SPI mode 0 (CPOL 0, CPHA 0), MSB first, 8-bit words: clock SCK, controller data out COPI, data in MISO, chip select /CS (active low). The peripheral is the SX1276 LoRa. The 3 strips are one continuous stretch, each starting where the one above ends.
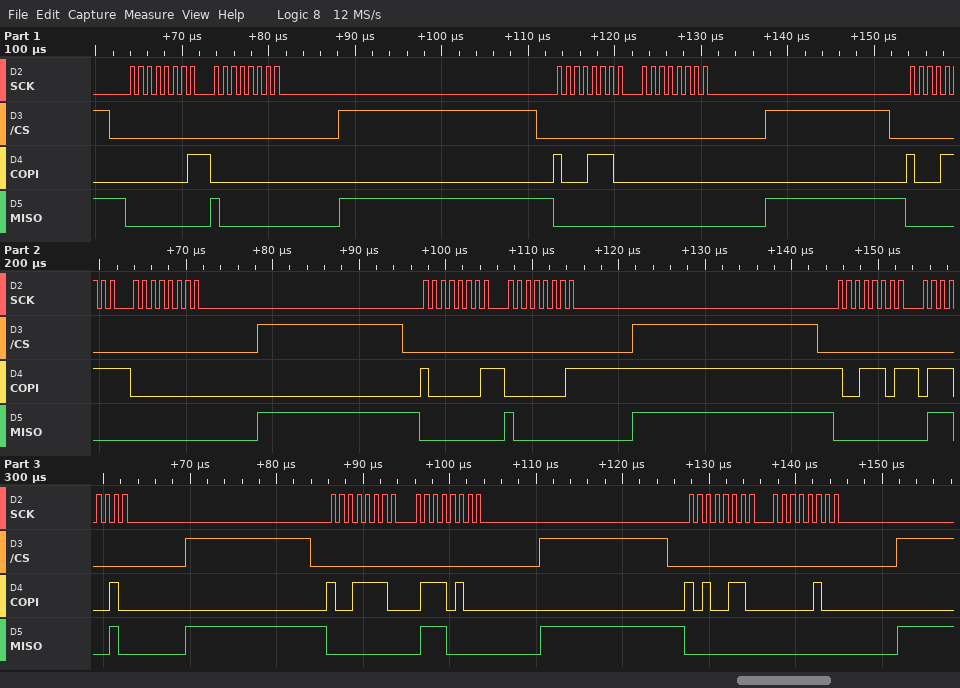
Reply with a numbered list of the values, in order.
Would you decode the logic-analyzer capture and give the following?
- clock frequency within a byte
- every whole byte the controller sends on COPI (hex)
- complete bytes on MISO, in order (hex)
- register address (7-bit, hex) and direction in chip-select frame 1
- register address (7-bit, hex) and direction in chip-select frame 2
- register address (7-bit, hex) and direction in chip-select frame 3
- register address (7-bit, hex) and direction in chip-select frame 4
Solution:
1. 1 MHz
2. 0x01 0x00 0x8E 0x00 0x8F 0x00 0x81 0x01 0x9D 0x72 0x9E 0x74 0xA6 0x04
3. 0x00 0x80 0x00 0x00 0x00 0x00 0x00 0x80 0x00 0x72 0x00 0x70 0x00 0x00
4. 0x01 read
5. 0x0E write
6. 0x0F write
7. 0x01 write
